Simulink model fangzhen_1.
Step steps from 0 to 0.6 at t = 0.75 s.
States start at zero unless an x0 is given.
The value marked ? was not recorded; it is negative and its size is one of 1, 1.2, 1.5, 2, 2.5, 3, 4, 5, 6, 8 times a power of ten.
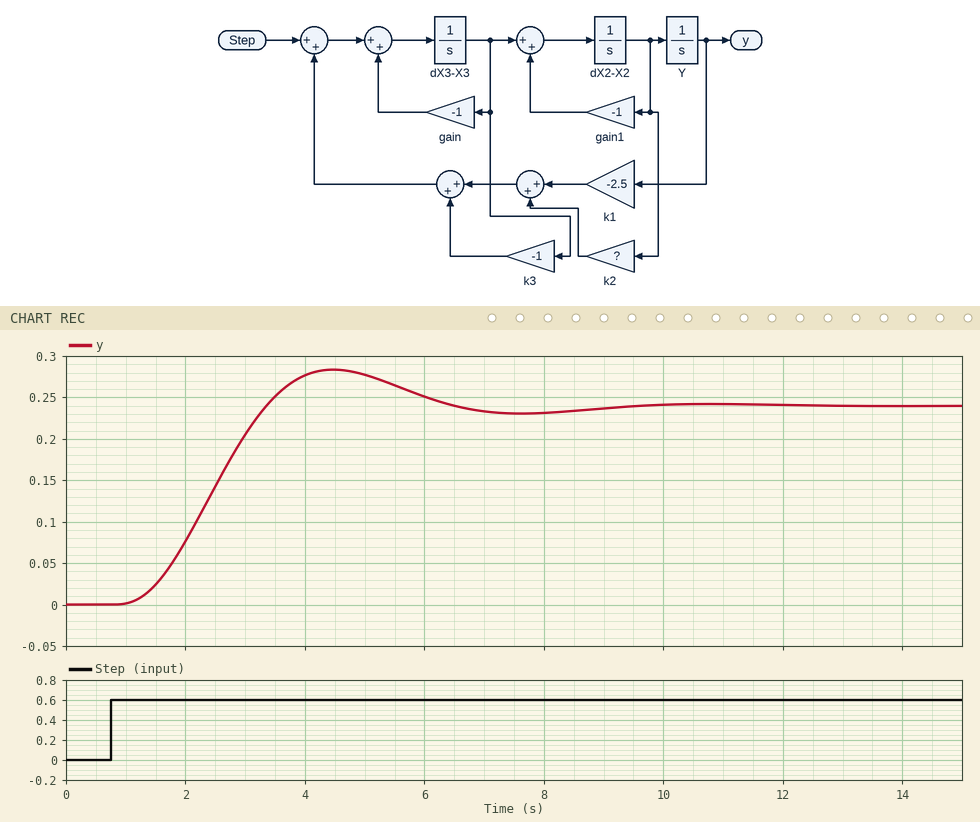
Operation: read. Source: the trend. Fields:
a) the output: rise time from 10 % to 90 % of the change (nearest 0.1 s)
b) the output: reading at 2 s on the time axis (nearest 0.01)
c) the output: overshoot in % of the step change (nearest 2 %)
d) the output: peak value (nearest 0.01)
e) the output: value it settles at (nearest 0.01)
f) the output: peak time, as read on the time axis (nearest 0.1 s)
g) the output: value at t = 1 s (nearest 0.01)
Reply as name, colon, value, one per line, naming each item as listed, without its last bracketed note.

the output: rise time from 10 % to 90 % of the change: 1.6 s
the output: reading at 2 s on the time axis: 0.08
the output: overshoot in % of the step change: 18 %
the output: peak value: 0.28
the output: value it settles at: 0.24
the output: peak time, as read on the time axis: 4.5 s
the output: value at t = 1 s: 0.00
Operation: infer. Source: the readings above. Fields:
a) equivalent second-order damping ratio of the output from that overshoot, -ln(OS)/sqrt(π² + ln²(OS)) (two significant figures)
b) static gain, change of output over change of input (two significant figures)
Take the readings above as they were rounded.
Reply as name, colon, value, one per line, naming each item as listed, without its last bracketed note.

equivalent second-order damping ratio of the output from that overshoot, -ln(OS)/sqrt(π² + ln²(OS)): 0.48
static gain, change of output over change of input: 0.40
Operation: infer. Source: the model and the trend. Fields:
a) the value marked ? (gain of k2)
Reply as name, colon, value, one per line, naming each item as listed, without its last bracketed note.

the value marked ?: -1.2
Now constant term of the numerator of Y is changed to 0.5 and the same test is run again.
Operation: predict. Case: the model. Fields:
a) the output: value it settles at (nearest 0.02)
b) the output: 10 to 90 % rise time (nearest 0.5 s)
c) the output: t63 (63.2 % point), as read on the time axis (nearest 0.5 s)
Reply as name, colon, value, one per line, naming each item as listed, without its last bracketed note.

the output: value it settles at: 0.24
the output: 10 to 90 % rise time: 3.5 s
the output: t63 (63.2 % point), as read on the time axis: 3.5 s
